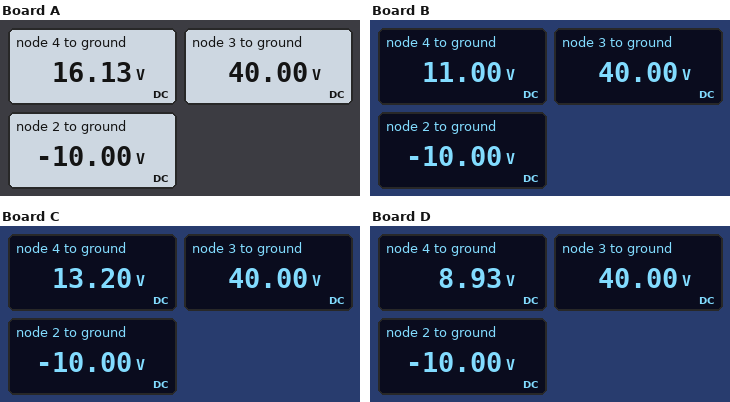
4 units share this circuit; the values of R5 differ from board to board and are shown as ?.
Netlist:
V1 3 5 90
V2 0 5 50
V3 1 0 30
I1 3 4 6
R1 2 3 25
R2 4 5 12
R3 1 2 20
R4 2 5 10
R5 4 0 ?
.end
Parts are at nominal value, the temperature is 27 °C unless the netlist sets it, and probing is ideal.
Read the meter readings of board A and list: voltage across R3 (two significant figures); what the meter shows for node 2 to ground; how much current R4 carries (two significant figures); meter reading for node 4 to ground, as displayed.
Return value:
40 V
-10.00 V
4.0 A
16.13 V
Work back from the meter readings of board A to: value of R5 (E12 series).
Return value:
33 Ω
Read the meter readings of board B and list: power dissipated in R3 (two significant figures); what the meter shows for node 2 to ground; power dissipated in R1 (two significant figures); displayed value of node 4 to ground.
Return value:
80 W
-10.00 V
100 W
11.00 V
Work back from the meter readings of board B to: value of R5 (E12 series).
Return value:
12 Ω
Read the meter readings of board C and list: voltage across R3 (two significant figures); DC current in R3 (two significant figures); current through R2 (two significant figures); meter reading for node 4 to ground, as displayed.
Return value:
40 V
2.0 A
5.3 A
13.20 V
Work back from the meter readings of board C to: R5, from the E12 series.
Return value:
18 Ω
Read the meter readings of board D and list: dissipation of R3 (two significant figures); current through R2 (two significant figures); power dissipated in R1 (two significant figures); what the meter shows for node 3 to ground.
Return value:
80 W
4.9 A
100 W
40.00 V
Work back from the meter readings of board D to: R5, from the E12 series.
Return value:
8.2 Ω
